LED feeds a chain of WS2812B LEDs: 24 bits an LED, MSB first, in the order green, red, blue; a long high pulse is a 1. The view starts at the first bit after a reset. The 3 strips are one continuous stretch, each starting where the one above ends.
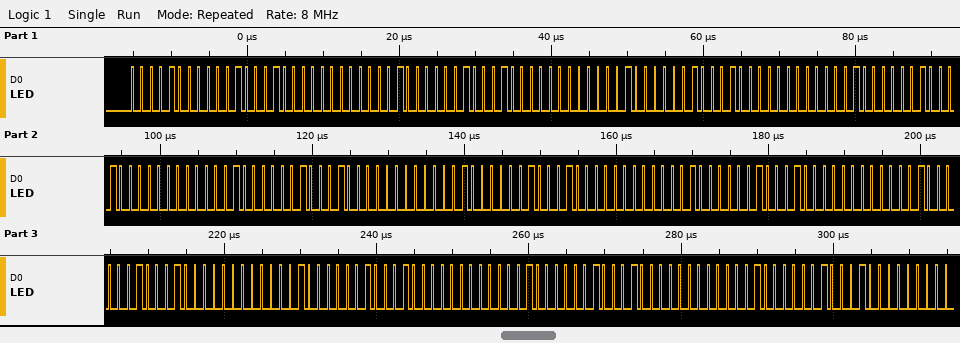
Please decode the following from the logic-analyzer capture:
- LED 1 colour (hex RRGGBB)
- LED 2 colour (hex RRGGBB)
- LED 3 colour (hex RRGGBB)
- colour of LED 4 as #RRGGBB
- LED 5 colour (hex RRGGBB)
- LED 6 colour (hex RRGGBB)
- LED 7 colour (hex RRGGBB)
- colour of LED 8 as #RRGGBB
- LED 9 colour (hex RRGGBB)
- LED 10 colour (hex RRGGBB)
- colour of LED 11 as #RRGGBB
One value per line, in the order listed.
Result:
#110800
#110800
#110800
#110800
#110800
#110800
#110800
#110800
#110800
#110800
#110800
